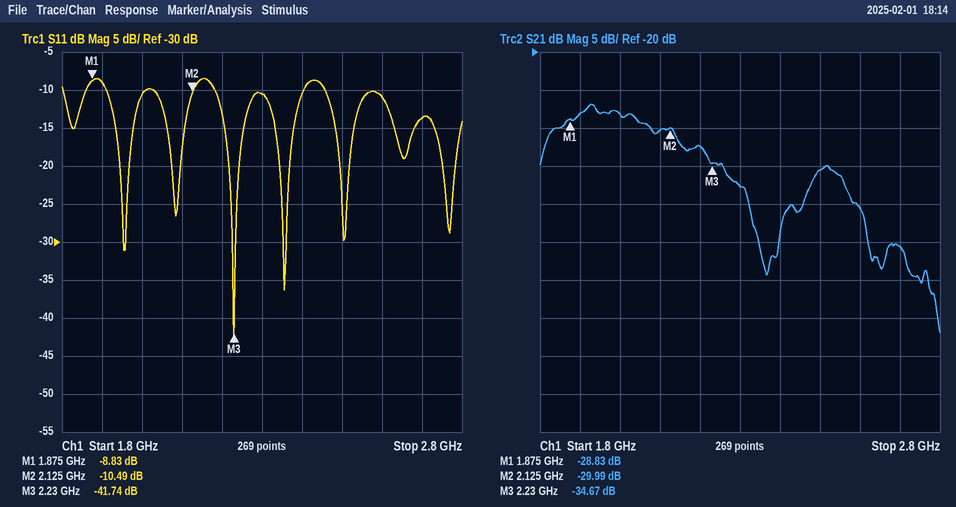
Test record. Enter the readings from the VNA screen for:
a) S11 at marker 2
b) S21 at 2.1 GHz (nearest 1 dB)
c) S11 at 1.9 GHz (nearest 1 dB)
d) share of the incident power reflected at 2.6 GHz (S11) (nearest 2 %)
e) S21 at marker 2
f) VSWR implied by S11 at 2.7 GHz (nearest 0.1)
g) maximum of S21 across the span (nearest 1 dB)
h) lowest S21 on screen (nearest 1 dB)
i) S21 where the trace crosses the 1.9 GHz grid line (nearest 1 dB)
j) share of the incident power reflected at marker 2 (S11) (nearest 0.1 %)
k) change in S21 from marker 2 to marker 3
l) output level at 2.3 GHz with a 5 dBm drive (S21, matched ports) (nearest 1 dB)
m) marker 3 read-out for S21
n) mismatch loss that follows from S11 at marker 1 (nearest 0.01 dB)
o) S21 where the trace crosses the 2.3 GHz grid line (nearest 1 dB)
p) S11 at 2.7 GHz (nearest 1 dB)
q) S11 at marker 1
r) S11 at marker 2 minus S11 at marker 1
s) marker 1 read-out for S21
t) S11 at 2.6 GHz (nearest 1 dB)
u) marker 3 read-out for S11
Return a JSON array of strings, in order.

["-10.49 dB", "-30 dB", "-9 dB", "8 %", "-29.99 dB", "1.5", "-27 dB", "-57 dB", "-28 dB", "8.9 %", "-4.68 dB", "-33 dBm", "-34.67 dB", "0.61 dB", "-38 dB", "-14 dB", "-8.83 dB", "-1.66 dB", "-28.83 dB", "-11 dB", "-41.74 dB"]
